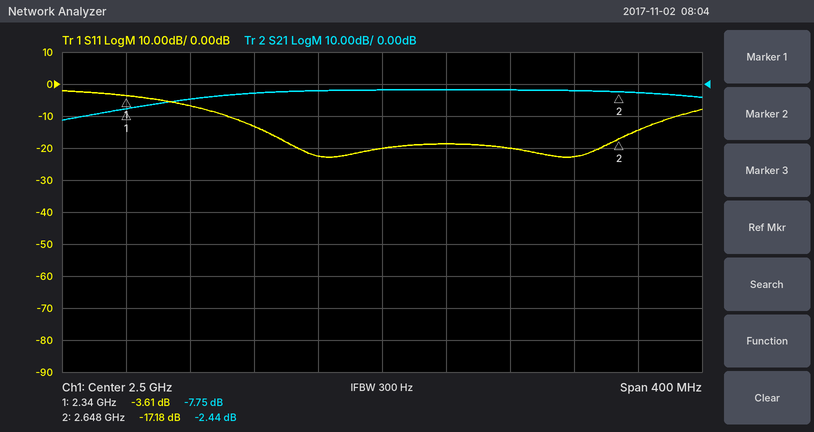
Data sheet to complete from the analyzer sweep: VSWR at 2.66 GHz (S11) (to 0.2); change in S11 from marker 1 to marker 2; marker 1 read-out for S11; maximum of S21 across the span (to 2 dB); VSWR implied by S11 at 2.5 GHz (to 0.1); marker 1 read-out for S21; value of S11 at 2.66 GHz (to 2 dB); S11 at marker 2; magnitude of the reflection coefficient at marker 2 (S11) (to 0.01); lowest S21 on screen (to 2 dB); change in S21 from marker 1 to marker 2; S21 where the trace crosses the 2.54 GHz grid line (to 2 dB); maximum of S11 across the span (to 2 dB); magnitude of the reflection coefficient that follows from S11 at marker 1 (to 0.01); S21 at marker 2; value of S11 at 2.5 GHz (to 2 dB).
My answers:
1.4
-13.57 dB
-3.61 dB
-2 dB
1.2
-7.75 dB
-14 dB
-17.18 dB
0.14
-12 dB
5.31 dB
-2 dB
-2 dB
0.66
-2.44 dB
-20 dB
